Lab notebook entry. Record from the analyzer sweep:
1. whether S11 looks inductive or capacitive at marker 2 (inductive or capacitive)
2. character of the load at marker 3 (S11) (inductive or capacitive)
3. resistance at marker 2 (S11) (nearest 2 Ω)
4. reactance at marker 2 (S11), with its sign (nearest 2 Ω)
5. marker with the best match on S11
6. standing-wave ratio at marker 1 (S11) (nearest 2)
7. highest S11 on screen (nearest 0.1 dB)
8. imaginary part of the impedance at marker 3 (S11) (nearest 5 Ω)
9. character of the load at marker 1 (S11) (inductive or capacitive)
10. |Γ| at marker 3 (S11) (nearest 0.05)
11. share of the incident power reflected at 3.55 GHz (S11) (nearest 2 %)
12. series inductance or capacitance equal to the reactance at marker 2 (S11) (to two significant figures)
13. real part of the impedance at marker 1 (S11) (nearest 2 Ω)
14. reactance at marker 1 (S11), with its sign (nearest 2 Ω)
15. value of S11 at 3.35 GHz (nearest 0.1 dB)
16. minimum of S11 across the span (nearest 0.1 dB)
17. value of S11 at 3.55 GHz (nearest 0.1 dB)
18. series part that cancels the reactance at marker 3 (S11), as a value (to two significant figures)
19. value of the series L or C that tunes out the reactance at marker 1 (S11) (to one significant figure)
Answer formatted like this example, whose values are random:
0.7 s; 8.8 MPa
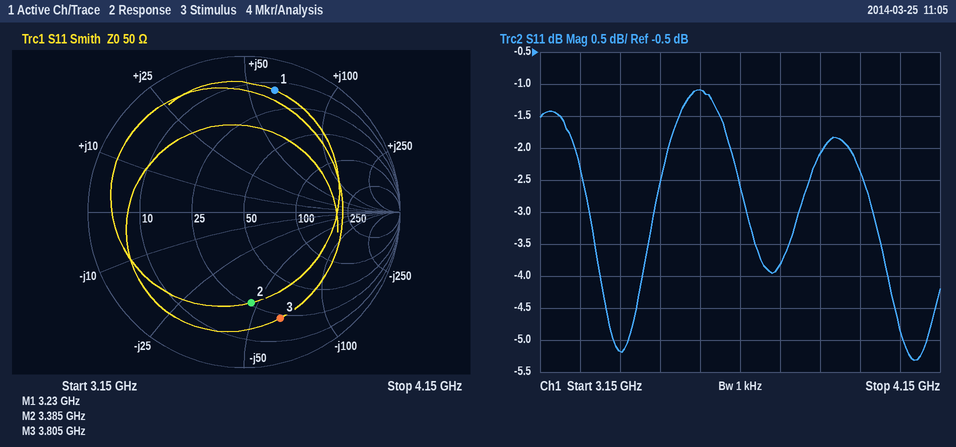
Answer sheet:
capacitive; capacitive; 26 Ω; -46 Ω; marker 2; 10; -1.1 dB; -65 Ω; inductive; 0.70; 78 %; 1.0 pF; 14 Ω; +62 Ω; -5.2 dB; -5.3 dB; -1.1 dB; 2.7 nH; 800 fF
